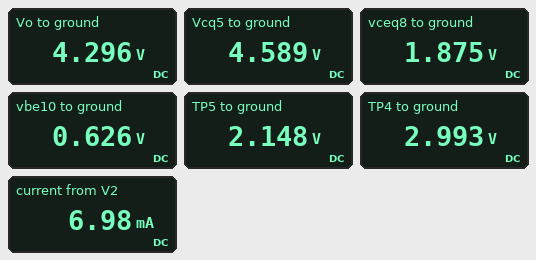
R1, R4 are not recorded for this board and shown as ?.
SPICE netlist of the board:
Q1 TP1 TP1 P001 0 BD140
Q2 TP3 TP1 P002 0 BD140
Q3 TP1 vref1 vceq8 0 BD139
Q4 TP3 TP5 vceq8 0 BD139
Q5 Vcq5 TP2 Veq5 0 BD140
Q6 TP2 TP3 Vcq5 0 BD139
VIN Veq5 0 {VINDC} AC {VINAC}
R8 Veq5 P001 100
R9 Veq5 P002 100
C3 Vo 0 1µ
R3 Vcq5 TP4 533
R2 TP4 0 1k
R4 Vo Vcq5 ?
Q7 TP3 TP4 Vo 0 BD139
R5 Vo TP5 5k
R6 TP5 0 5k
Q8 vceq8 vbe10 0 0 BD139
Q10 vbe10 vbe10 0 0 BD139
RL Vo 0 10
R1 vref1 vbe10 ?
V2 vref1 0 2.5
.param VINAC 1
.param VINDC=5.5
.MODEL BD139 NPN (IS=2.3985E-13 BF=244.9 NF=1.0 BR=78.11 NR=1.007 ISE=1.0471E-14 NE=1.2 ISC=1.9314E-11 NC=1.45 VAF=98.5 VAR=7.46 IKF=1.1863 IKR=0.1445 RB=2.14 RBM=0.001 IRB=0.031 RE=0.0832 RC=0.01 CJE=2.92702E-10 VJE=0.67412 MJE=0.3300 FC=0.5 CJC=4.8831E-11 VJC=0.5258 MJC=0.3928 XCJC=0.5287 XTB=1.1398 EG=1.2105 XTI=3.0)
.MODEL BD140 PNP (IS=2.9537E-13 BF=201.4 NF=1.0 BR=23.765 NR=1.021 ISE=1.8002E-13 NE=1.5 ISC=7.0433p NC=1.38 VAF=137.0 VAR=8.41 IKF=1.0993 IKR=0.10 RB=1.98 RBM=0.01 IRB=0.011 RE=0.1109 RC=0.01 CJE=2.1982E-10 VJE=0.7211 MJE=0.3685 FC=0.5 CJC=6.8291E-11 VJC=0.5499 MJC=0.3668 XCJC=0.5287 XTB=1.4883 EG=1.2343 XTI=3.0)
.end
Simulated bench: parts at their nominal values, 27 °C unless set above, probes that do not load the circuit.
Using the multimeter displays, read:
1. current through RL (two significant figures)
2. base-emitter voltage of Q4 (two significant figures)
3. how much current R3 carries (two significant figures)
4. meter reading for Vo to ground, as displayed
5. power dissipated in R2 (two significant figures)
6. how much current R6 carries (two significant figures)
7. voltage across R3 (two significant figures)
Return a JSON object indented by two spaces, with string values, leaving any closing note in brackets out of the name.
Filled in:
{
  "current through RL": "430 mA",
  "base-emitter voltage of Q4": "270 mV",
  "how much current R3 carries": "3.0 mA",
  "meter reading for Vo to ground, as displayed": "4.296 V",
  "power dissipated in R2": "9.0 mW",
  "how much current R6 carries": "430 µA",
  "voltage across R3": "1.6 V"
}
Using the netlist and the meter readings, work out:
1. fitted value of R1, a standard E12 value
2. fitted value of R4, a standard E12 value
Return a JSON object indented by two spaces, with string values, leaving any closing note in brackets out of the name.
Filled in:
{
  "fitted value of R1, a standard E12 value": "270 Ω",
  "fitted value of R4, a standard E12 value": "0.68 Ω"
}
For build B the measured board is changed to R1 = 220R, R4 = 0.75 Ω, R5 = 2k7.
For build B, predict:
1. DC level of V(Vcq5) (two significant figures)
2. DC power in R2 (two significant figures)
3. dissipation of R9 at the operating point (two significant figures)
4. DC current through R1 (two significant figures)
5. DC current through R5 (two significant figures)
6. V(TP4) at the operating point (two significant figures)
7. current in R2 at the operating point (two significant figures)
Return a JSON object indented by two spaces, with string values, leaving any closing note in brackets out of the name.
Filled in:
{
  "DC level of V(Vcq5)": "4.2 V",
  "DC power in R2": "7.5 mW",
  "dissipation of R9 at the operating point": "1.8 mW",
  "DC current through R1": "8.5 mA",
  "DC current through R5": "520 µA",
  "V(TP4) at the operating point": "2.7 V",
  "current in R2 at the operating point": "2.7 mA"
}
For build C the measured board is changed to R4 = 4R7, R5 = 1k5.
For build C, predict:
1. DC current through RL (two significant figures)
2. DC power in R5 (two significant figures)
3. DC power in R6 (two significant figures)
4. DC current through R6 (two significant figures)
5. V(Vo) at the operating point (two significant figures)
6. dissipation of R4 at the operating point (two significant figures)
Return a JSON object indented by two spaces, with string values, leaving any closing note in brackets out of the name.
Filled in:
{
  "DC current through RL": "310 mA",
  "DC power in R5": "350 µW",
  "DC power in R6": "1.2 mW",
  "DC current through R6": "480 µA",
  "V(Vo) at the operating point": "3.1 V",
  "dissipation of R4 at the operating point": "460 mW"
}
